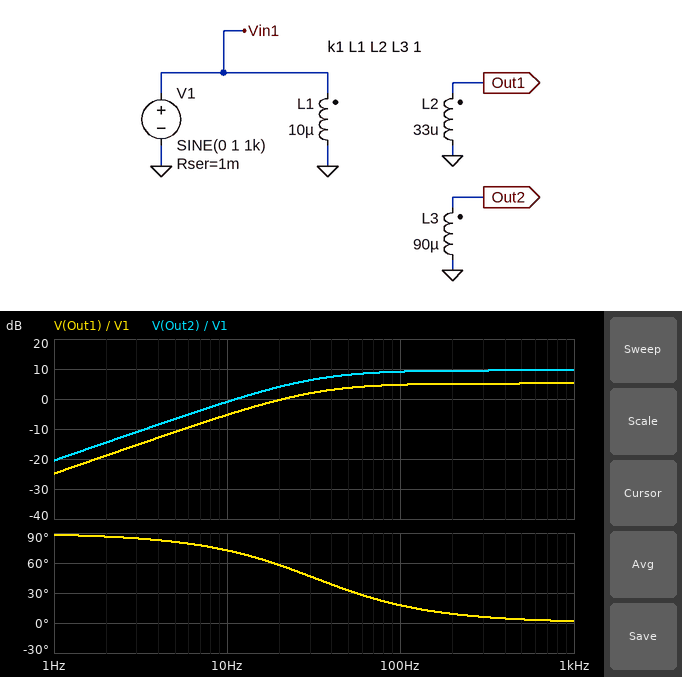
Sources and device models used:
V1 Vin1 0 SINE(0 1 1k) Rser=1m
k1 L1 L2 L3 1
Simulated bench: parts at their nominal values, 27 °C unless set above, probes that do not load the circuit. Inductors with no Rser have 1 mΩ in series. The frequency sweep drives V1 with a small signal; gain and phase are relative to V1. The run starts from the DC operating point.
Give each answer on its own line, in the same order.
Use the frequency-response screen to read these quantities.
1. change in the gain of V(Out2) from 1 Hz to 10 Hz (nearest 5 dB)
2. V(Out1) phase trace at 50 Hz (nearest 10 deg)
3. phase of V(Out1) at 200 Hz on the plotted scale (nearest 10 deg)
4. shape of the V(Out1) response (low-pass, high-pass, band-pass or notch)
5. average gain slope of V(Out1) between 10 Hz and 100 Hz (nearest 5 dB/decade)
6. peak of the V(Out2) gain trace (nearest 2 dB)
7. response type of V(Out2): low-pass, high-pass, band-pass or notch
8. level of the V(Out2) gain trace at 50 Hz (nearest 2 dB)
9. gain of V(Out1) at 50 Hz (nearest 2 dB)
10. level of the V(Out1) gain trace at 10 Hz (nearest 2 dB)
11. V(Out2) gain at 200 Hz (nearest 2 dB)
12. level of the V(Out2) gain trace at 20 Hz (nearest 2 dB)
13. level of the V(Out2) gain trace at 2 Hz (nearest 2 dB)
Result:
20 dB
30 deg
10 deg
high-pass
10 dB/decade
10 dB
high-pass
8 dB
4 dB
-6 dB
10 dB
4 dB
-14 dB
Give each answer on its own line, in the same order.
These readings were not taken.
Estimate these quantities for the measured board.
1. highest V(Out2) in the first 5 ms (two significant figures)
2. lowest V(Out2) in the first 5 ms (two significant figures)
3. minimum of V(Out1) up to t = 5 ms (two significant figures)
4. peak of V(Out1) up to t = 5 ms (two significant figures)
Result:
3.0 V
-3.1 V
-1.9 V
1.8 V
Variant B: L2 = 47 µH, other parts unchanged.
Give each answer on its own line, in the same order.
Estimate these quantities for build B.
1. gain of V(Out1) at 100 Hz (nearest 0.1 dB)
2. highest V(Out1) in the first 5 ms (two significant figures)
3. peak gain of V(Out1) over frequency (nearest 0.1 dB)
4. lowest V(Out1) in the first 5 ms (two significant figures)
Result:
6.3 dB
2.1 V
6.7 dB
-2.2 V
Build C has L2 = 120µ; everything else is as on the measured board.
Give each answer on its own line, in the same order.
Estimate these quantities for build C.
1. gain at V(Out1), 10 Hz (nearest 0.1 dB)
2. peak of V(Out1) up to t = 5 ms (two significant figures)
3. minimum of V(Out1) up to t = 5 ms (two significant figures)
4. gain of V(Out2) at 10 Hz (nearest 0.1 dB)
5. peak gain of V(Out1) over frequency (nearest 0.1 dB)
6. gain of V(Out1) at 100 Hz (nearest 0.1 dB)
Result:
0.3 dB
3.4 V
-3.6 V
-0.9 dB
10.8 dB
10.4 dB
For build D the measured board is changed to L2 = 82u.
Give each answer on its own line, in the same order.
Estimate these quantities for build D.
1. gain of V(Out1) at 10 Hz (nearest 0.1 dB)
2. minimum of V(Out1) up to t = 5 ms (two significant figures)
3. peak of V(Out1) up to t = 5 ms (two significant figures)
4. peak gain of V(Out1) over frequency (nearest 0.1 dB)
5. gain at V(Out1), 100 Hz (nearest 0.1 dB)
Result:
-1.3 dB
-2.9 V
2.8 V
9.1 dB
8.7 dB
